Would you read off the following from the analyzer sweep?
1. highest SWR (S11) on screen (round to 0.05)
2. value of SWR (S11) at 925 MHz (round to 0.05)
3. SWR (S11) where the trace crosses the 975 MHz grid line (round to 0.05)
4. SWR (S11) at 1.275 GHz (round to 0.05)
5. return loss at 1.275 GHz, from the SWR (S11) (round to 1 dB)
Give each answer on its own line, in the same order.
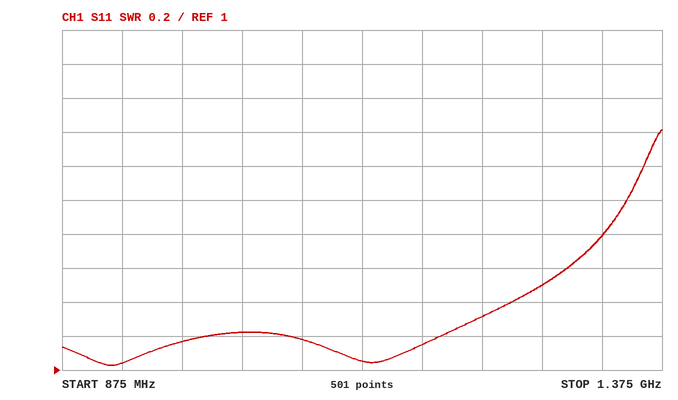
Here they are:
2.40
1.05
1.15
1.50
14 dB
